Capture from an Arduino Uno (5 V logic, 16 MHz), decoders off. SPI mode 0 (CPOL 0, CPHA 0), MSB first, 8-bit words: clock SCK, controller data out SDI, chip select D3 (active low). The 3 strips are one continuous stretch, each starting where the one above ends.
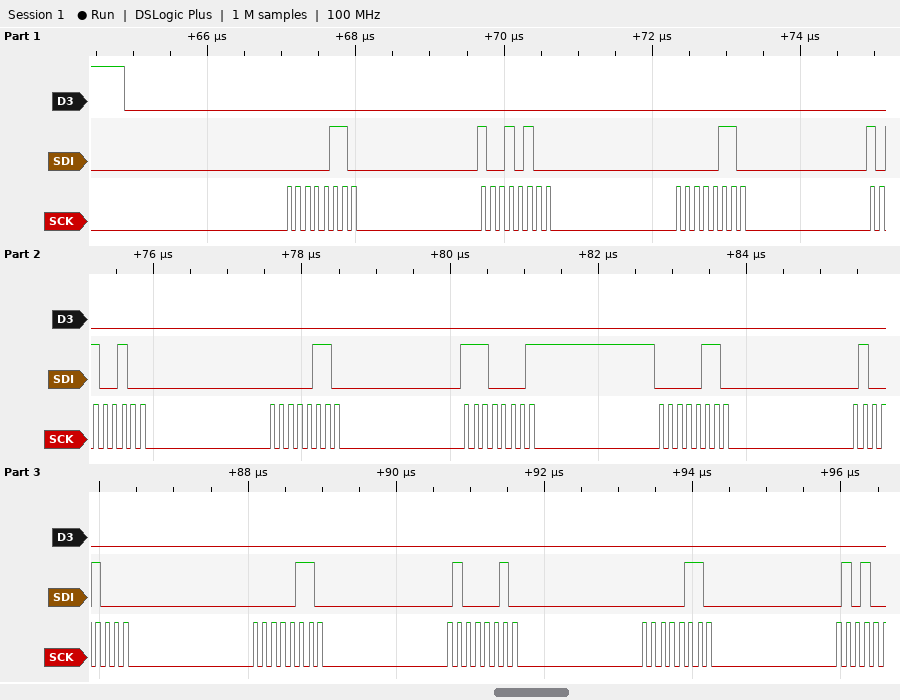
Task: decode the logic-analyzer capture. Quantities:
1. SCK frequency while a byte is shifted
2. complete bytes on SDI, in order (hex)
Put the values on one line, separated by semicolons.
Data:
8 MHz; 0x06 0x94 0x06 0xA4 0x06 0xE1 0x06 0x48 0x06 0x42 0x06
